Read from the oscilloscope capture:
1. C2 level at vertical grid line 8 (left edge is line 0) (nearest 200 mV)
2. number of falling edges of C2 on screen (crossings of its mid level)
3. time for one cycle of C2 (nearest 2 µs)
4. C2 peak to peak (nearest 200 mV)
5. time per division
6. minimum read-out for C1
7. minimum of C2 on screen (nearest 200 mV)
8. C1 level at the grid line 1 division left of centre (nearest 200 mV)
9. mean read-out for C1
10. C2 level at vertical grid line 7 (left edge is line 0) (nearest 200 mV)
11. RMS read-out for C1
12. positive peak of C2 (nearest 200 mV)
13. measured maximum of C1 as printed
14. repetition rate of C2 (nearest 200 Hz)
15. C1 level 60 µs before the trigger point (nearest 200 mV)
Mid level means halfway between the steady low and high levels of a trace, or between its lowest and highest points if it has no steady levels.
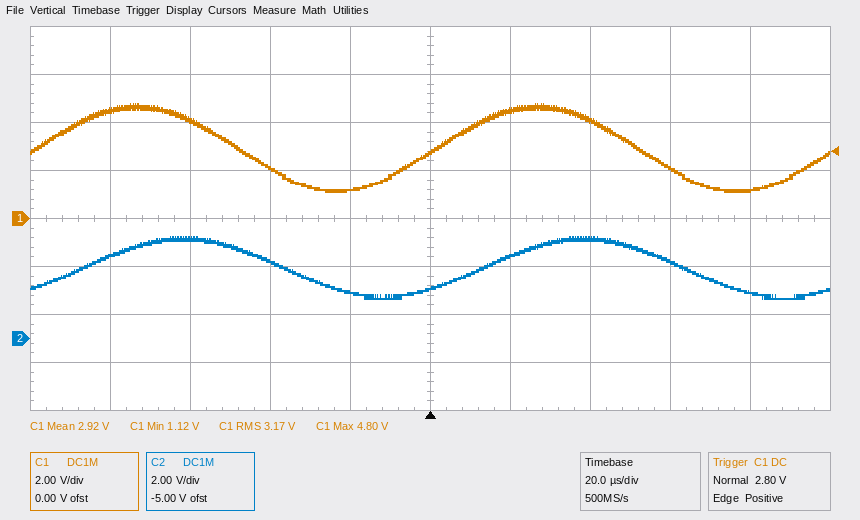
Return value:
3.2 V
2
100 µs
2.6 V
20 µs
1.12 V
1.6 V
1.2 V
2.92 V
4.2 V
3.17 V
4.2 V
4.80 V
10.0 kHz
4.0 V
